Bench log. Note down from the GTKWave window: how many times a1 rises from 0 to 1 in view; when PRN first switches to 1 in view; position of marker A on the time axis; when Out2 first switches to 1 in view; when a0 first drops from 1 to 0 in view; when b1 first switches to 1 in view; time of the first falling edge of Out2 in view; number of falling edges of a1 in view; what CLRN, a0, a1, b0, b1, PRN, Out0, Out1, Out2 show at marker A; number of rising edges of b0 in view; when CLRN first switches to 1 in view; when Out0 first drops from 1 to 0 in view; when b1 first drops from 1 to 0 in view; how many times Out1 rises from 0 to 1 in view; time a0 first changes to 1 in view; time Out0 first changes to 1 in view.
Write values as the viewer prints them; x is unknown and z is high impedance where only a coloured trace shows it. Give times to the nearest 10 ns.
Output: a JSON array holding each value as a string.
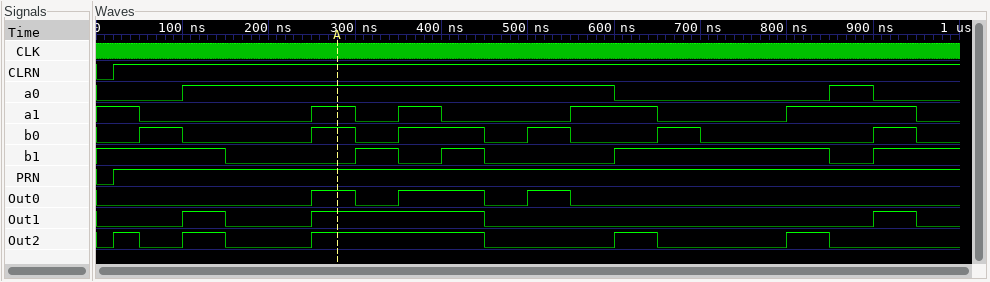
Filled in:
["4", "20 ns", "280 ns", "20 ns", "600 ns", "300 ns", "50 ns", "5", "CLRN=1, a0=1, a1=1, b0=1, b1=0, PRN=1, Out0=1, Out1=1, Out2=1", "6", "20 ns", "300 ns", "150 ns", "3", "100 ns", "250 ns"]
